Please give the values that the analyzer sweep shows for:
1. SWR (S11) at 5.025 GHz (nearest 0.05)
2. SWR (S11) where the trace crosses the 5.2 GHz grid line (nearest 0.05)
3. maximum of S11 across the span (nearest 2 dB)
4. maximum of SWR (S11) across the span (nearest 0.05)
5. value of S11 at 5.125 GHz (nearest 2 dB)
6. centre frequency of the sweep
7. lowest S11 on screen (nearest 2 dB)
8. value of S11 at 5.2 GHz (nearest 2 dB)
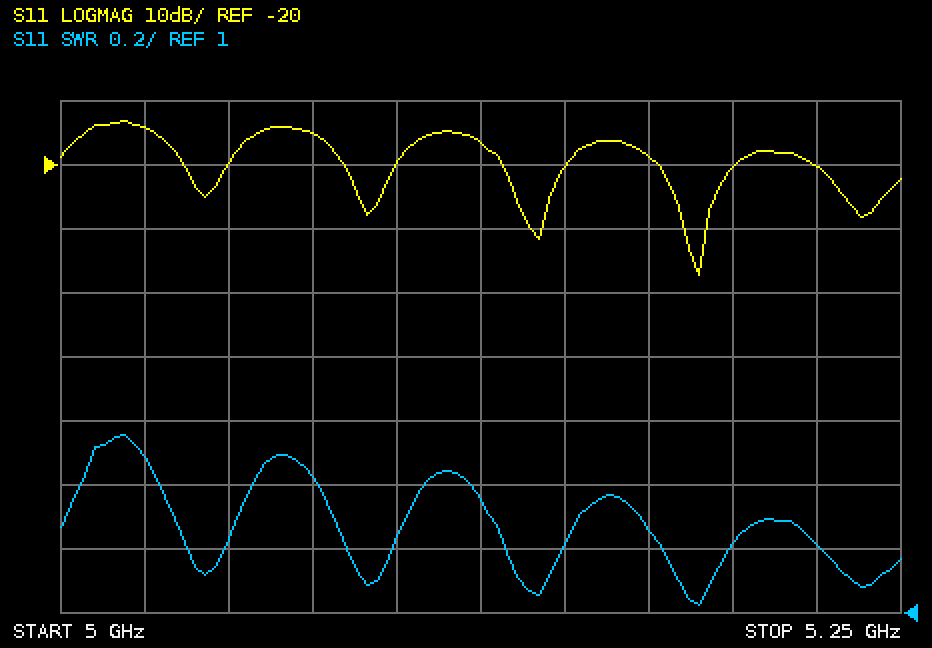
1.50
1.20
-14 dB
1.55
-16 dB
5.125 GHz
-38 dB
-20 dB
